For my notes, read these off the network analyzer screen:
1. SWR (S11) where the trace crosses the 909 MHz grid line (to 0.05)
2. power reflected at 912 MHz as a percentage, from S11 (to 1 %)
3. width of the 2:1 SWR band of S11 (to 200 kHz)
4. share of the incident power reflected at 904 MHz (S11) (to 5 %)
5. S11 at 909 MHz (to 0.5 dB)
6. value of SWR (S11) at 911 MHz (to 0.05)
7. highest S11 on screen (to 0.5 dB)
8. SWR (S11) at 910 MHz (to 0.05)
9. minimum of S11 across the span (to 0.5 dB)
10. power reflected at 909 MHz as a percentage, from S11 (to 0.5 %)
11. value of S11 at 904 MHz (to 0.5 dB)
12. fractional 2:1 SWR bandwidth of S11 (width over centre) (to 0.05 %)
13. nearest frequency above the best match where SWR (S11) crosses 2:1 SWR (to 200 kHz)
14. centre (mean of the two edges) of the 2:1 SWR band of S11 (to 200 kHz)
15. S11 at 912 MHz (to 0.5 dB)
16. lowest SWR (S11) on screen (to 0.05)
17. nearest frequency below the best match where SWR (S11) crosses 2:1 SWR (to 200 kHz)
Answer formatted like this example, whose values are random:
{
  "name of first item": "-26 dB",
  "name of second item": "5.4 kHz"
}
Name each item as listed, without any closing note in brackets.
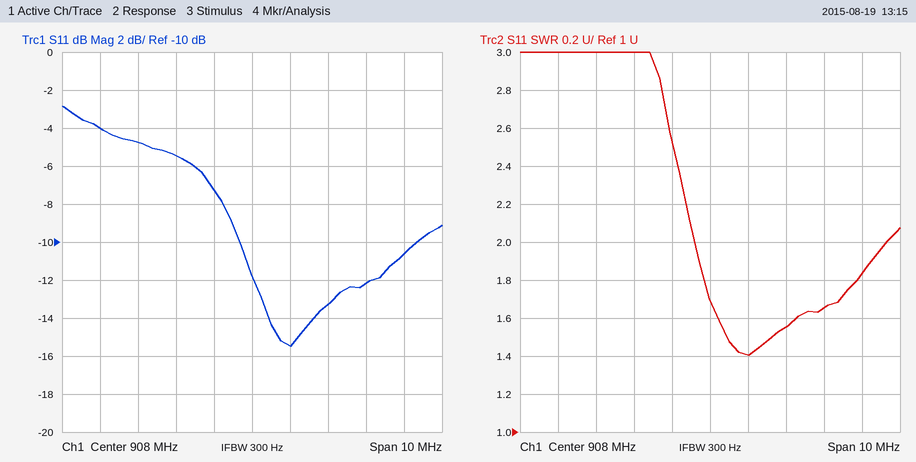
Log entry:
{
  "SWR (S11) where the trace crosses the 909 MHz grid line": "1.40",
  "power reflected at 912 MHz as a percentage, from S11": "9 %",
  "width of the 2:1 SWR band of S11": "5.0 MHz",
  "share of the incident power reflected at 904 MHz (S11)": "40 %",
  "S11 at 909 MHz": "-15.5 dB",
  "value of SWR (S11) at 911 MHz": "1.65",
  "highest S11 on screen": "-3.0 dB",
  "SWR (S11) at 910 MHz": "1.55",
  "minimum of S11 across the span": "-15.5 dB",
  "power reflected at 909 MHz as a percentage, from S11": "3.0 %",
  "value of S11 at 904 MHz": "-4.0 dB",
  "fractional 2:1 SWR bandwidth of S11 (width over centre)": "0.55 %",
  "nearest frequency above the best match where SWR (S11) crosses 2:1 SWR": "912.6 MHz",
  "centre (mean of the two edges) of the 2:1 SWR band of S11": "910.2 MHz",
  "S11 at 912 MHz": "-10.5 dB",
  "lowest SWR (S11) on screen": "1.40",
  "nearest frequency below the best match where SWR (S11) crosses 2:1 SWR": "907.6 MHz"
}
